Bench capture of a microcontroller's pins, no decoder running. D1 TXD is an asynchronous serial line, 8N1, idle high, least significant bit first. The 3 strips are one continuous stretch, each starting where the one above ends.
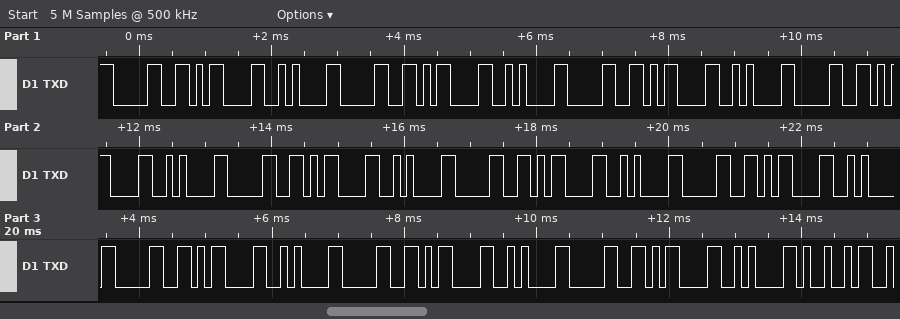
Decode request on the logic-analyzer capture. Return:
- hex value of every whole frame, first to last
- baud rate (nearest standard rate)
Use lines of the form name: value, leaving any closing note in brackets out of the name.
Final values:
hex value of every whole frame, first to last: 0x30 0x0D 0x0A 0x30 0x0D 0x0A 0x30 0x0D 0x0A 0x30 0x0D 0x0A 0x30 0x0D 0x0A 0x30 0x0D 0x0A 0x30 0x0D 0x0A 0x30 0x0D 0x0A 0x30 0x0D 0x0A 0x30 0x0D 0x0A 0x49
baud rate: 9600 baud
